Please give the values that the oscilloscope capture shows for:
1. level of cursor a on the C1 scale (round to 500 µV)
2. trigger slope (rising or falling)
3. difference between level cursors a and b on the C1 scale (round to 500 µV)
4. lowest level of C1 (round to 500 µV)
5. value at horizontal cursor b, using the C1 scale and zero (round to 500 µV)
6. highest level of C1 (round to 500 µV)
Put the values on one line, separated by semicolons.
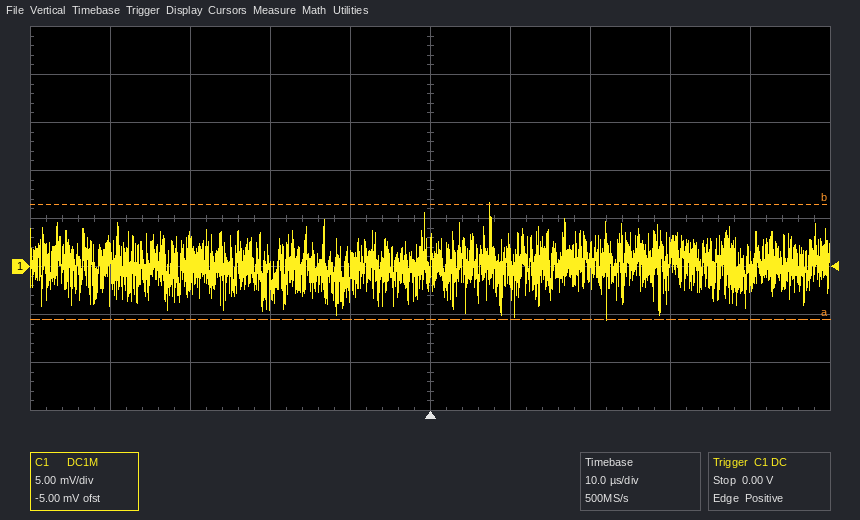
-5.5 mV; rising; 12.0 mV; -5.5 mV; 6.5 mV; 6.5 mV
